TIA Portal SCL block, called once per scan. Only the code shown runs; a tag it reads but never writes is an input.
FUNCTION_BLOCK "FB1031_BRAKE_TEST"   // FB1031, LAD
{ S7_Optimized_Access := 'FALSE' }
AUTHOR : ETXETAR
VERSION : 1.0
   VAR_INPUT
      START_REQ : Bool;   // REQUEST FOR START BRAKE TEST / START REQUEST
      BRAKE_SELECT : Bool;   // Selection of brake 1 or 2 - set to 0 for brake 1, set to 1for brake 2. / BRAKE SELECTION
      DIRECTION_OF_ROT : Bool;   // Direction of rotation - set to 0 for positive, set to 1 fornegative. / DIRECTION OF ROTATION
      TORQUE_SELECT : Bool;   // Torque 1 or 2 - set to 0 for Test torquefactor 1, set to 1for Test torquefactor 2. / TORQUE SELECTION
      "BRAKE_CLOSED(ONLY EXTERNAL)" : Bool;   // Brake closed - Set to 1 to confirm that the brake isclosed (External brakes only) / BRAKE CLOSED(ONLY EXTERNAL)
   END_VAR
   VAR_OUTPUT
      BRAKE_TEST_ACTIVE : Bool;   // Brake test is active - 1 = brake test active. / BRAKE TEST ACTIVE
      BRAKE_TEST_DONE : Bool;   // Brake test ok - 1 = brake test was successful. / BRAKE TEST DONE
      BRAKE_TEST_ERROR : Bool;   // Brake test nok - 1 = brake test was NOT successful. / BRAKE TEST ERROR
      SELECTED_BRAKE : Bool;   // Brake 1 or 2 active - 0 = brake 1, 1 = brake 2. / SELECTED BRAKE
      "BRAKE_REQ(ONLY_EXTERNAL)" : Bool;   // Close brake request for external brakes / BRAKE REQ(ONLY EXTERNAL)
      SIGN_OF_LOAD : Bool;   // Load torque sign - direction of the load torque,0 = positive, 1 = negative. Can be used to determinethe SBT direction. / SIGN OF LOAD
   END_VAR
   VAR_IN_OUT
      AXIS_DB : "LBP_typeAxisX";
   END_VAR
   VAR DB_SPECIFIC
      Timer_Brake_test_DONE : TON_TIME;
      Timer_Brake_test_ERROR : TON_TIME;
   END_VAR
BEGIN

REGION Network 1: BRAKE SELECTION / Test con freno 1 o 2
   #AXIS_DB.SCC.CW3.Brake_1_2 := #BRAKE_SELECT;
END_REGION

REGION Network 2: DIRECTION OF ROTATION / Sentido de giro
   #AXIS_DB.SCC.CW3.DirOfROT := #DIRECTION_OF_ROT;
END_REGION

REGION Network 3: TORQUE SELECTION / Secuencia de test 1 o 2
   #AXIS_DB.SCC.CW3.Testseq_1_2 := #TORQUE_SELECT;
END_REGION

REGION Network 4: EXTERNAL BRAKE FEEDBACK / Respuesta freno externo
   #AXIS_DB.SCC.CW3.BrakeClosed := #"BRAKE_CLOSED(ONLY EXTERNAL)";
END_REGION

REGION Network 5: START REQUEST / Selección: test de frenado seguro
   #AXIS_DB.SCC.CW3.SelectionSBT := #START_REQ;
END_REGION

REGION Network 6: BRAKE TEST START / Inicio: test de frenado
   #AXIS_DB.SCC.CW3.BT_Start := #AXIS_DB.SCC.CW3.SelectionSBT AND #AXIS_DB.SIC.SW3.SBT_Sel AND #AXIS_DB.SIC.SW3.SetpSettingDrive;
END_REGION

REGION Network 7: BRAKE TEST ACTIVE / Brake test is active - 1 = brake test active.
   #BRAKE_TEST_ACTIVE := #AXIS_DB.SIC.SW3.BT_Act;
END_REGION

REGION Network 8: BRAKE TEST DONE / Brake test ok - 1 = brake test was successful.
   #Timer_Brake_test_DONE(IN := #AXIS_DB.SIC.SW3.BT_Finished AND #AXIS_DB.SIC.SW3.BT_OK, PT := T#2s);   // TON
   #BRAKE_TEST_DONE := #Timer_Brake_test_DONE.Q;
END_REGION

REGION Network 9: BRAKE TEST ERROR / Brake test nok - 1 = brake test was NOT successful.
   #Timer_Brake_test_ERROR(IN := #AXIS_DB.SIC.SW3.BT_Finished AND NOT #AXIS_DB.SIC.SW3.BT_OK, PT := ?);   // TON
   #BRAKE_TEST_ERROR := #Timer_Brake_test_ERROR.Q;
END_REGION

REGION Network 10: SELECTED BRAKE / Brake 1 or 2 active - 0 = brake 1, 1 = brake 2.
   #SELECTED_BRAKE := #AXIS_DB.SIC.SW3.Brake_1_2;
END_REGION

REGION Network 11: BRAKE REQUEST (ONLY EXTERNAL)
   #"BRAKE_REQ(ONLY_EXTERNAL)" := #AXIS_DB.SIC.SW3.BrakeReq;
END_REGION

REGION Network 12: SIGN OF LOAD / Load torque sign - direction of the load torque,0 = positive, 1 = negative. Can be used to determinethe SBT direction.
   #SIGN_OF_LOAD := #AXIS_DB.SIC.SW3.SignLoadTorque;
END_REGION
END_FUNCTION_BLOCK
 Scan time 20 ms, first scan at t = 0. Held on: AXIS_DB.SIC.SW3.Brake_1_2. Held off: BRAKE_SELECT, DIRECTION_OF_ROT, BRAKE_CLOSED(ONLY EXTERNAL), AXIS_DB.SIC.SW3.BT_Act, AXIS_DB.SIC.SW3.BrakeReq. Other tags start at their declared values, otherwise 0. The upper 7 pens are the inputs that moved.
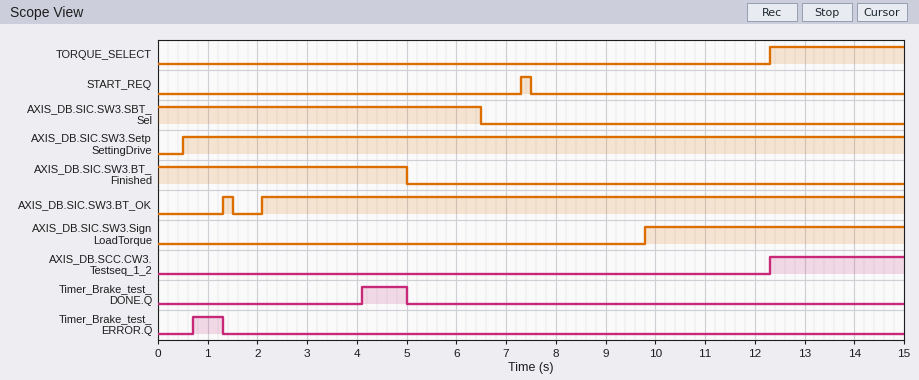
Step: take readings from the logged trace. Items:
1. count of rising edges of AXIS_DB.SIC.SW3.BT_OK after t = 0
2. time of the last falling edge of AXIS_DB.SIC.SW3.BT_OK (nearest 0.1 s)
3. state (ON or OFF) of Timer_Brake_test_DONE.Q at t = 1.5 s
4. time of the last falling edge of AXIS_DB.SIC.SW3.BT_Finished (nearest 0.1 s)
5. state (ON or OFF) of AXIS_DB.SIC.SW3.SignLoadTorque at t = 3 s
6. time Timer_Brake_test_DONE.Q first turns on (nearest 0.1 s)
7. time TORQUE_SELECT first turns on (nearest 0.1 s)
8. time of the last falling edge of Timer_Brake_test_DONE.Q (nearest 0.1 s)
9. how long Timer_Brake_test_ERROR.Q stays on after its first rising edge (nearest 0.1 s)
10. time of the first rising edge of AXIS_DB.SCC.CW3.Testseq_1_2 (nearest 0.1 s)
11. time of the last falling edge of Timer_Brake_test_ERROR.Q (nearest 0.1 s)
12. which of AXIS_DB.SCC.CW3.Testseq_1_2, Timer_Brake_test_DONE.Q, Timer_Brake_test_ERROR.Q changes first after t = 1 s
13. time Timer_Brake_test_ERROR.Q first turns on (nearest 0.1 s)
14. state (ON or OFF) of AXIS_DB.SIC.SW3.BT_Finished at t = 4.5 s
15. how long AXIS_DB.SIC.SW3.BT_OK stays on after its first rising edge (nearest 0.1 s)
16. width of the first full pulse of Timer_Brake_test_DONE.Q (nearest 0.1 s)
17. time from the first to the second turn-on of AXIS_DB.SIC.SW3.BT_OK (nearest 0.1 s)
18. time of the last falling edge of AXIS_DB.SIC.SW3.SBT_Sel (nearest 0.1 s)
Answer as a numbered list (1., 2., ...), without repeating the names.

1. 2
2. 1.5 s
3. OFF
4. 5.0 s
5. OFF
6. 4.1 s
7. 12.3 s
8. 5.0 s
9. 0.6 s
10. 12.3 s
11. 1.3 s
12. Timer_Brake_test_ERROR.Q
13. 0.7 s
14. ON
15. 0.2 s
16. 0.9 s
17. 0.8 s
18. 6.5 s
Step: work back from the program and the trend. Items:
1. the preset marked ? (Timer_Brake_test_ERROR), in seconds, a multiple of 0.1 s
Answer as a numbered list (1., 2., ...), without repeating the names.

1. 0.7 s
